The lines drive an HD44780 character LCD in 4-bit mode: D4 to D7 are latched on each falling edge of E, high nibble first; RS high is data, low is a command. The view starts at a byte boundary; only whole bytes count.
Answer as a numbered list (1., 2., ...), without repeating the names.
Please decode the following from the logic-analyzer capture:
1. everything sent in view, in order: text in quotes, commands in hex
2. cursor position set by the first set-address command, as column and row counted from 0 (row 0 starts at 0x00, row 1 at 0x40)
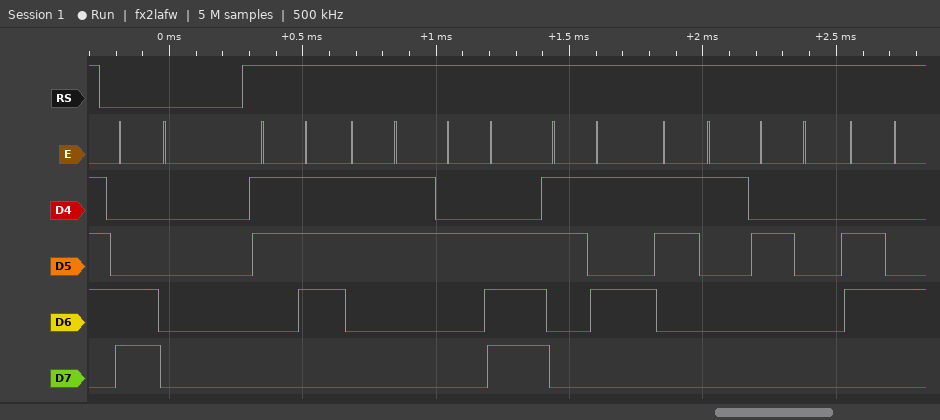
1. 0xC0 "73.51 d"
2. column 0, row 1
